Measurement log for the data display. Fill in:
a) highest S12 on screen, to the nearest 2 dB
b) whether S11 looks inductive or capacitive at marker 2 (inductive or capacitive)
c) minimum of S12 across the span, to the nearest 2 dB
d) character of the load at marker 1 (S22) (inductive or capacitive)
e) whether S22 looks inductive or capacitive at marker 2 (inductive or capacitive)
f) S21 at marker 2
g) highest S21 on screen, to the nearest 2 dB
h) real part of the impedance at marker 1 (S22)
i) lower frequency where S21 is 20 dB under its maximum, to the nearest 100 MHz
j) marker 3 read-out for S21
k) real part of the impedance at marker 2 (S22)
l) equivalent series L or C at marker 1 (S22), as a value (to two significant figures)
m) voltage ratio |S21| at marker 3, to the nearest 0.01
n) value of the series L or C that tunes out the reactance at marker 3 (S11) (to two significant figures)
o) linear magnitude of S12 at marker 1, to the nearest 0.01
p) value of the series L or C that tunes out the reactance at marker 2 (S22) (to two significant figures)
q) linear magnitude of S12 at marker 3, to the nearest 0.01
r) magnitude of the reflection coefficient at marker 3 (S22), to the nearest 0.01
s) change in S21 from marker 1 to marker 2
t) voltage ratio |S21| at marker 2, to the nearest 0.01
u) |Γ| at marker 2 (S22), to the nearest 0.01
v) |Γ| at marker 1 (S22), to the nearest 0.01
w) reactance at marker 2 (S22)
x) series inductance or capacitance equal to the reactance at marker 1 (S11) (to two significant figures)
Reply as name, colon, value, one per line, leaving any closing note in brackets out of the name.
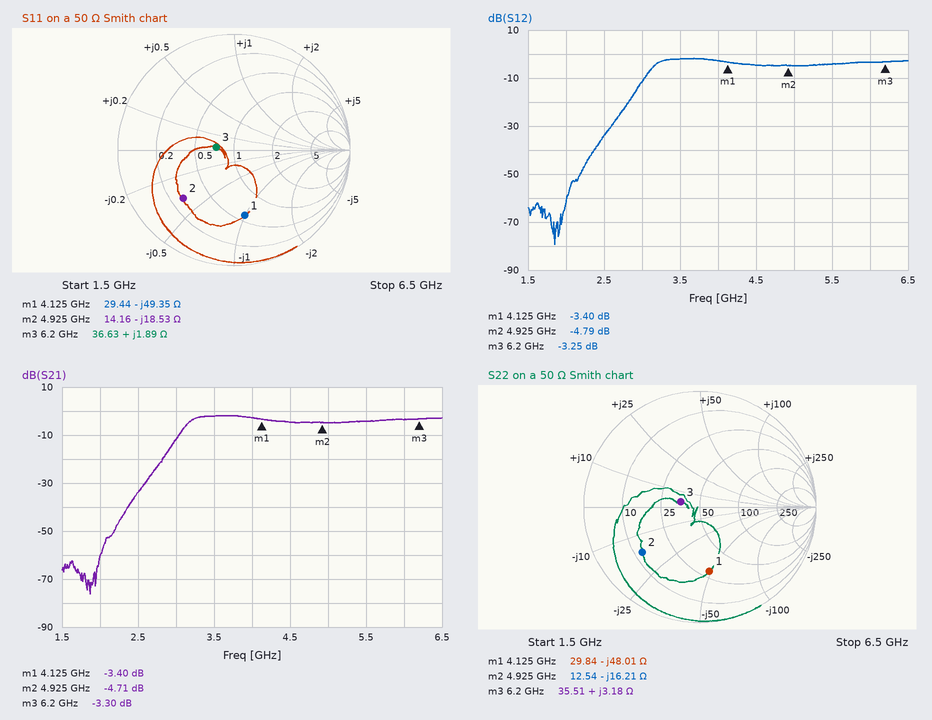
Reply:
highest S12 on screen, to the nearest 2 dB: -2 dB
whether S11 looks inductive or capacitive at marker 2: capacitive
minimum of S12 across the span, to the nearest 2 dB: -80 dB
character of the load at marker 1 (S22): capacitive
whether S22 looks inductive or capacitive at marker 2: capacitive
S21 at marker 2: -4.71 dB
highest S21 on screen, to the nearest 2 dB: -2 dB
real part of the impedance at marker 1: 29.84 Ω
lower frequency where S21 is 20 dB under its maximum, to the nearest 100 MHz: 2.8 GHz
marker 3 read-out for S21: -3.30 dB
real part of the impedance at marker 2: 12.54 Ω
equivalent series L or C at marker 1 (S22), as a value: 800 fF
voltage ratio |S21| at marker 3, to the nearest 0.01: 0.68
value of the series L or C that tunes out the reactance at marker 3 (S11): 14 pF
linear magnitude of S12 at marker 1, to the nearest 0.01: 0.68
value of the series L or C that tunes out the reactance at marker 2 (S22): 520 pH
linear magnitude of S12 at marker 3, to the nearest 0.01: 0.69
magnitude of the reflection coefficient at marker 3 (S22), to the nearest 0.01: 0.17
change in S21 from marker 1 to marker 2: -1.31 dB
voltage ratio |S21| at marker 2, to the nearest 0.01: 0.58
|Γ| at marker 2 (S22), to the nearest 0.01: 0.63
|Γ| at marker 1 (S22), to the nearest 0.01: 0.56
reactance at marker 2: -16.21 Ω
series inductance or capacitance equal to the reactance at marker 1 (S11): 780 fF
